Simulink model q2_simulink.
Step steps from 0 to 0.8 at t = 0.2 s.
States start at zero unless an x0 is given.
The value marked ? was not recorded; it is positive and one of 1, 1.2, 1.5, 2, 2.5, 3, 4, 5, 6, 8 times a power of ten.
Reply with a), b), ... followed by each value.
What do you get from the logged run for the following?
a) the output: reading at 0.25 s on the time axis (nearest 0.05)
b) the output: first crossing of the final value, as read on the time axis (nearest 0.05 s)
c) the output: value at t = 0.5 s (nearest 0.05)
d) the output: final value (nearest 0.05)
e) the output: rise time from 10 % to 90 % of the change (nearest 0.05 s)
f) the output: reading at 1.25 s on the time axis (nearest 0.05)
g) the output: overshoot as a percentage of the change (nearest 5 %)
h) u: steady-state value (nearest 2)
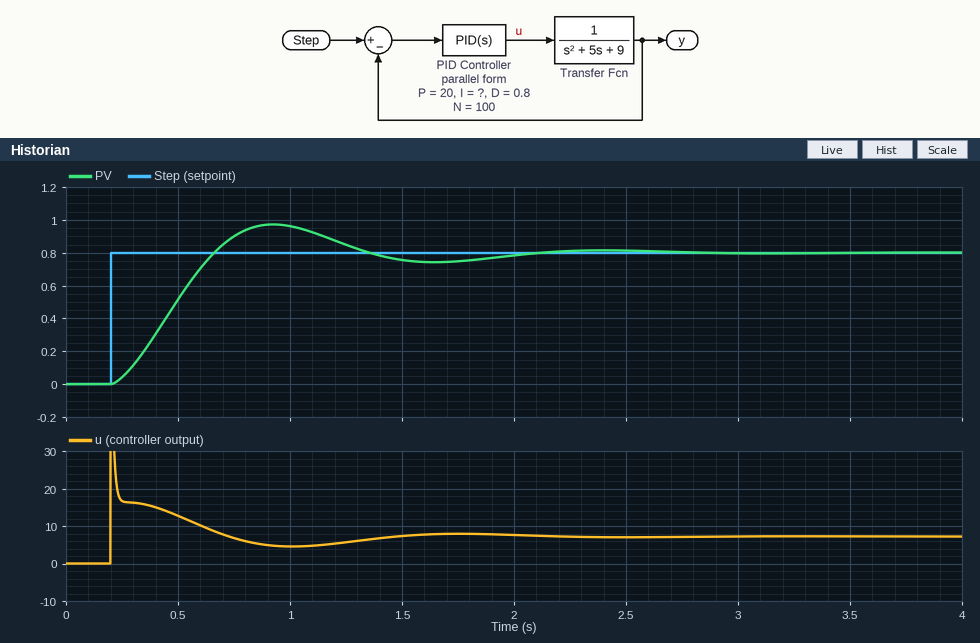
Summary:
a) 0.05
b) 0.65 s
c) 0.50
d) 0.80
e) 0.35 s
f) 0.85
g) 20 %
h) 8
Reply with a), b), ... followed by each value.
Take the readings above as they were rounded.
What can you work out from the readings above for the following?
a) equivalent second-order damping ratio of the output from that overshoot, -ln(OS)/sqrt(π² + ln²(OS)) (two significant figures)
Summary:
a) 0.46
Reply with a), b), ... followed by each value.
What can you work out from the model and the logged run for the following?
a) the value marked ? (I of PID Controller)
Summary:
a) 50
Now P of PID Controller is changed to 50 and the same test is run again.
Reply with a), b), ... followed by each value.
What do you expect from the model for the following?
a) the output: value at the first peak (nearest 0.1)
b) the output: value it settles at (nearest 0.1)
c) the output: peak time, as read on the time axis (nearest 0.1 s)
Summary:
a) 1.0
b) 0.8
c) 0.6 s
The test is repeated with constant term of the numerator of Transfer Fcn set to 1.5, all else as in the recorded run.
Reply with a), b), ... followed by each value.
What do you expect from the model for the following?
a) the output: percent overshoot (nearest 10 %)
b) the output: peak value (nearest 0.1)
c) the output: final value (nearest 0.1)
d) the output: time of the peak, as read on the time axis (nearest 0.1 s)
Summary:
a) 30 %
b) 1.0
c) 0.8
d) 0.8 s
